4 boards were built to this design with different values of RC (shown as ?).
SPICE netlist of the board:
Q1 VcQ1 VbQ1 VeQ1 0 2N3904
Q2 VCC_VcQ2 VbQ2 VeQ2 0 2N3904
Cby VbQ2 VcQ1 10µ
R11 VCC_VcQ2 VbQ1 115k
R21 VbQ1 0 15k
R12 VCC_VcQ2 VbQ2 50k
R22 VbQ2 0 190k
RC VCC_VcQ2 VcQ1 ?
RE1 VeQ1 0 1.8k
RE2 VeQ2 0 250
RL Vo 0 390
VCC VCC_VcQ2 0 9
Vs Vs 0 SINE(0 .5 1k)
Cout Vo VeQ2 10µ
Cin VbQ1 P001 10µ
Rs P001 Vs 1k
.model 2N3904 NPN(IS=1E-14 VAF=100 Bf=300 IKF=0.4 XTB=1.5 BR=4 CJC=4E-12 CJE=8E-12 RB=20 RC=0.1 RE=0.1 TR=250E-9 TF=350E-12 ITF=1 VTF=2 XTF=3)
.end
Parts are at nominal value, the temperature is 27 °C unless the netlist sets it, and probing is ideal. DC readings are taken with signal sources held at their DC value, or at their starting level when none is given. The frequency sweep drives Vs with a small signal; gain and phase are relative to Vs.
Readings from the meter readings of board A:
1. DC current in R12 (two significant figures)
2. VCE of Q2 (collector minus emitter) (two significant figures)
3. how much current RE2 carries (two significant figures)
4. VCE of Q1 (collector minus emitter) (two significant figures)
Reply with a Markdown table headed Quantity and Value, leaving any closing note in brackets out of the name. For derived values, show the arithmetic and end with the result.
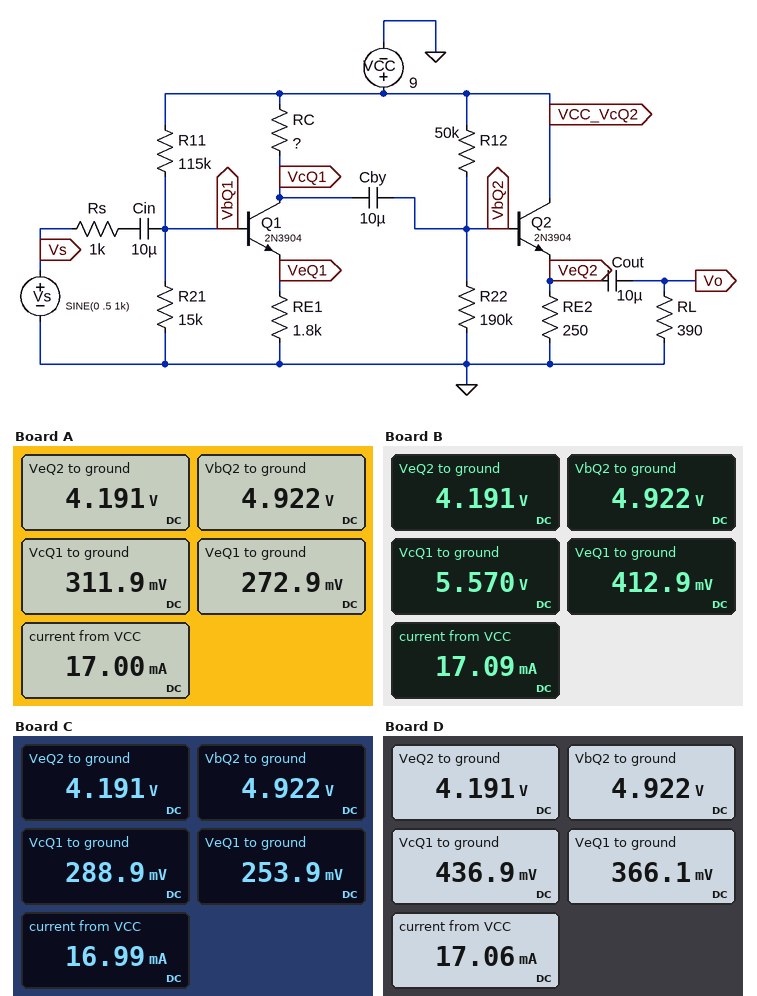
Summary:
| Quantity | Value |
|---|---|
| DC current in R12 | (9 V - 4.922 V) / 50 kΩ = 82 µA |
| VCE of Q2 (collector minus emitter) | 9 V - 4.191 V = 4.8 V |
| how much current RE2 carries | (4.191 V) / 250 Ω = 17 mA |
| VCE of Q1 (collector minus emitter) | 311.9 mV - 272.9 mV = 39 mV |
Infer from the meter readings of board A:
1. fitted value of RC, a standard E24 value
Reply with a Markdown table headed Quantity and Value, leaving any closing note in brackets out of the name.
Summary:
| Quantity | Value |
|---|---|
| fitted value of RC, a standard E24 value | 62 kΩ |
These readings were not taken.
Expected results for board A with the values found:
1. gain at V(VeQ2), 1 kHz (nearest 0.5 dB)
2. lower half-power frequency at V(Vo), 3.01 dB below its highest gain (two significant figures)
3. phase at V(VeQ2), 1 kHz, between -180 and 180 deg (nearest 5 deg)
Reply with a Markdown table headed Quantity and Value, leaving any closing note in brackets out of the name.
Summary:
| Quantity | Value |
|---|---|
| gain at V(VeQ2), 1 kHz | -32.0 dB |
| lower half-power frequency at V(Vo), 3.01 dB below its highest gain | 200 kHz |
| phase at V(VeQ2), 1 kHz, between -180 and 180 deg | 5 deg |
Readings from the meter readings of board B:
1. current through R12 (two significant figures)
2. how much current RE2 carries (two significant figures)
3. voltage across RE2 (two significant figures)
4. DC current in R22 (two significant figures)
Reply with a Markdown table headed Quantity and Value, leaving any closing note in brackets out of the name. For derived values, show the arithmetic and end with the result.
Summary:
| Quantity | Value |
|---|---|
| current through R12 | (9 V - 4.922 V) / 50 kΩ = 82 µA |
| how much current RE2 carries | (4.191 V) / 250 Ω = 17 mA |
| voltage across RE2 | 4.191 V = 4.2 V |
| DC current in R22 | (4.922 V) / 190 kΩ = 26 µA |
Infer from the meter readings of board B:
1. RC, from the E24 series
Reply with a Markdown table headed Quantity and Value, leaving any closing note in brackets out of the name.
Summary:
| Quantity | Value |
|---|---|
| RC, from the E24 series | 15 kΩ |
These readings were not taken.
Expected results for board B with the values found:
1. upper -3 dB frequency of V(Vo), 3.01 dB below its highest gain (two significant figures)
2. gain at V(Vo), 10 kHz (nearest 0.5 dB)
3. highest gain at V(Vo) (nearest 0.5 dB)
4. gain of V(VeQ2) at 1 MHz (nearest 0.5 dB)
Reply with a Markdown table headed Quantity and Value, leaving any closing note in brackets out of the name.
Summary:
| Quantity | Value |
|---|---|
| upper -3 dB frequency of V(Vo), 3.01 dB below its highest gain | 2.3 MHz |
| gain at V(Vo), 10 kHz | 12.5 dB |
| highest gain at V(Vo) | 12.5 dB |
| gain of V(VeQ2) at 1 MHz | 11.5 dB |
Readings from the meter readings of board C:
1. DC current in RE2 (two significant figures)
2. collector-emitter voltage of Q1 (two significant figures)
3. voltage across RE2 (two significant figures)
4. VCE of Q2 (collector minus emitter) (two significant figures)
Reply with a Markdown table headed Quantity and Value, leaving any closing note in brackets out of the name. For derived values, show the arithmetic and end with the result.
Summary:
| Quantity | Value |
|---|---|
| DC current in RE2 | (4.191 V) / 250 Ω = 17 mA |
| collector-emitter voltage of Q1 | 288.9 mV - 253.9 mV = 35 mV |
| voltage across RE2 | 4.191 V = 4.2 V |
| VCE of Q2 (collector minus emitter) | 9 V - 4.191 V = 4.8 V |
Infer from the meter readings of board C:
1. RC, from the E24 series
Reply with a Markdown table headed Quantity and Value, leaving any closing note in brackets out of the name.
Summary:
| Quantity | Value |
|---|---|
| RC, from the E24 series | 68 kΩ |
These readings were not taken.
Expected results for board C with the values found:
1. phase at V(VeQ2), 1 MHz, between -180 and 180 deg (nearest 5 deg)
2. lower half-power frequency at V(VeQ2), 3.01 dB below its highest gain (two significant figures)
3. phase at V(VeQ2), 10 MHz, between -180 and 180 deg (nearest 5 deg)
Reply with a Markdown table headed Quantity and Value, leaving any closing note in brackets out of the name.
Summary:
| Quantity | Value |
|---|---|
| phase at V(VeQ2), 1 MHz, between -180 and 180 deg | 10 deg |
| lower half-power frequency at V(VeQ2), 3.01 dB below its highest gain | 190 kHz |
| phase at V(VeQ2), 10 MHz, between -180 and 180 deg | -10 deg |
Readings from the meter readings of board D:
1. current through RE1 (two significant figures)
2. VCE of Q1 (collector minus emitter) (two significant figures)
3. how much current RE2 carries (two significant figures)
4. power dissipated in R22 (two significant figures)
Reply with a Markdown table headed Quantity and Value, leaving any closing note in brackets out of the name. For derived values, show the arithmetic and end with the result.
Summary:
| Quantity | Value |
|---|---|
| current through RE1 | (366.1 mV) / 1.8 kΩ = 200 µA |
| VCE of Q1 (collector minus emitter) | 436.9 mV - 366.1 mV = 71 mV |
| how much current RE2 carries | (4.191 V) / 250 Ω = 17 mA |
| power dissipated in R22 | (4.922 V)^2 / 190 kΩ = 130 µW |
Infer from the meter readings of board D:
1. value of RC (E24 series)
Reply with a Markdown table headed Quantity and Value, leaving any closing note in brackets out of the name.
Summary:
| Quantity | Value |
|---|---|
| value of RC | 43 kΩ |
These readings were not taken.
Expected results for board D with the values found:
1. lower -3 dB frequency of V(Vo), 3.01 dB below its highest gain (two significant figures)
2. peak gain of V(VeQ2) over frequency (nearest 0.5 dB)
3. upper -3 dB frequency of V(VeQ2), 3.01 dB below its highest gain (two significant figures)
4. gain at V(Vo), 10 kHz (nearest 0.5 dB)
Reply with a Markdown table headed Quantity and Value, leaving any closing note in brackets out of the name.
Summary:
| Quantity | Value |
|---|---|
| lower -3 dB frequency of V(Vo), 3.01 dB below its highest gain | 40 Hz |
| peak gain of V(VeQ2) over frequency | 0 dB |
| upper -3 dB frequency of V(VeQ2), 3.01 dB below its highest gain | 380 kHz |
| gain at V(Vo), 10 kHz | 0 dB |
